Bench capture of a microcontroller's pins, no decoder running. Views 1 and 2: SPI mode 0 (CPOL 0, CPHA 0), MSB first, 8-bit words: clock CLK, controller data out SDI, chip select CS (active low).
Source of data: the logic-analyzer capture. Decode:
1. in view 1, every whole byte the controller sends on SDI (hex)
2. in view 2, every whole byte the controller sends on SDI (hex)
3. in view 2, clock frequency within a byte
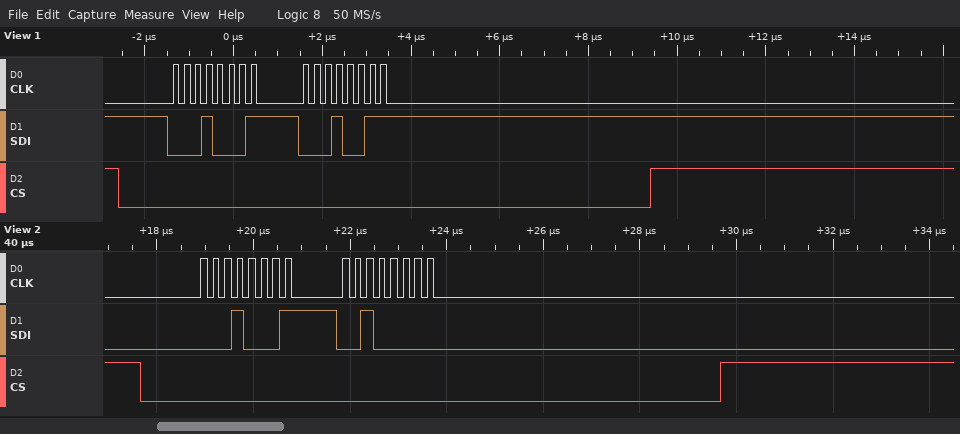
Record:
11 13
11 20
4 MHz
